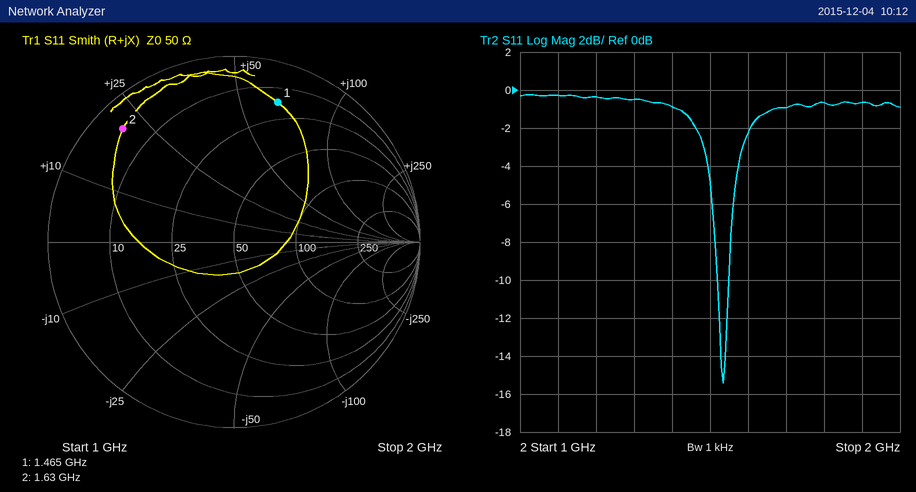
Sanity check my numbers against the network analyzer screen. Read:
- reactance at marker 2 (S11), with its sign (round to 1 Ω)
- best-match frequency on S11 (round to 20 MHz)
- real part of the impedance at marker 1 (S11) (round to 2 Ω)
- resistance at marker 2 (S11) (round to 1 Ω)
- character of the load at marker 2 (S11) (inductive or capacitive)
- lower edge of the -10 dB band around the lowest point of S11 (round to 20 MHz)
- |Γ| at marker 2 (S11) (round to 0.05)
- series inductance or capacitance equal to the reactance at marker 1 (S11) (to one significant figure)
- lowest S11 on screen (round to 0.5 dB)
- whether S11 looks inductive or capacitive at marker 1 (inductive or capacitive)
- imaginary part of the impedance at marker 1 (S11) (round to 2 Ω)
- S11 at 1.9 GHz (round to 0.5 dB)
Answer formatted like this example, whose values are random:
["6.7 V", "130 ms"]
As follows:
["+21 Ω", "1.54 GHz", "16 Ω", "5 Ω", "inductive", "1.52 GHz", "0.85", "7 nH", "-15.5 dB", "inductive", "+66 Ω", "-0.5 dB"]
